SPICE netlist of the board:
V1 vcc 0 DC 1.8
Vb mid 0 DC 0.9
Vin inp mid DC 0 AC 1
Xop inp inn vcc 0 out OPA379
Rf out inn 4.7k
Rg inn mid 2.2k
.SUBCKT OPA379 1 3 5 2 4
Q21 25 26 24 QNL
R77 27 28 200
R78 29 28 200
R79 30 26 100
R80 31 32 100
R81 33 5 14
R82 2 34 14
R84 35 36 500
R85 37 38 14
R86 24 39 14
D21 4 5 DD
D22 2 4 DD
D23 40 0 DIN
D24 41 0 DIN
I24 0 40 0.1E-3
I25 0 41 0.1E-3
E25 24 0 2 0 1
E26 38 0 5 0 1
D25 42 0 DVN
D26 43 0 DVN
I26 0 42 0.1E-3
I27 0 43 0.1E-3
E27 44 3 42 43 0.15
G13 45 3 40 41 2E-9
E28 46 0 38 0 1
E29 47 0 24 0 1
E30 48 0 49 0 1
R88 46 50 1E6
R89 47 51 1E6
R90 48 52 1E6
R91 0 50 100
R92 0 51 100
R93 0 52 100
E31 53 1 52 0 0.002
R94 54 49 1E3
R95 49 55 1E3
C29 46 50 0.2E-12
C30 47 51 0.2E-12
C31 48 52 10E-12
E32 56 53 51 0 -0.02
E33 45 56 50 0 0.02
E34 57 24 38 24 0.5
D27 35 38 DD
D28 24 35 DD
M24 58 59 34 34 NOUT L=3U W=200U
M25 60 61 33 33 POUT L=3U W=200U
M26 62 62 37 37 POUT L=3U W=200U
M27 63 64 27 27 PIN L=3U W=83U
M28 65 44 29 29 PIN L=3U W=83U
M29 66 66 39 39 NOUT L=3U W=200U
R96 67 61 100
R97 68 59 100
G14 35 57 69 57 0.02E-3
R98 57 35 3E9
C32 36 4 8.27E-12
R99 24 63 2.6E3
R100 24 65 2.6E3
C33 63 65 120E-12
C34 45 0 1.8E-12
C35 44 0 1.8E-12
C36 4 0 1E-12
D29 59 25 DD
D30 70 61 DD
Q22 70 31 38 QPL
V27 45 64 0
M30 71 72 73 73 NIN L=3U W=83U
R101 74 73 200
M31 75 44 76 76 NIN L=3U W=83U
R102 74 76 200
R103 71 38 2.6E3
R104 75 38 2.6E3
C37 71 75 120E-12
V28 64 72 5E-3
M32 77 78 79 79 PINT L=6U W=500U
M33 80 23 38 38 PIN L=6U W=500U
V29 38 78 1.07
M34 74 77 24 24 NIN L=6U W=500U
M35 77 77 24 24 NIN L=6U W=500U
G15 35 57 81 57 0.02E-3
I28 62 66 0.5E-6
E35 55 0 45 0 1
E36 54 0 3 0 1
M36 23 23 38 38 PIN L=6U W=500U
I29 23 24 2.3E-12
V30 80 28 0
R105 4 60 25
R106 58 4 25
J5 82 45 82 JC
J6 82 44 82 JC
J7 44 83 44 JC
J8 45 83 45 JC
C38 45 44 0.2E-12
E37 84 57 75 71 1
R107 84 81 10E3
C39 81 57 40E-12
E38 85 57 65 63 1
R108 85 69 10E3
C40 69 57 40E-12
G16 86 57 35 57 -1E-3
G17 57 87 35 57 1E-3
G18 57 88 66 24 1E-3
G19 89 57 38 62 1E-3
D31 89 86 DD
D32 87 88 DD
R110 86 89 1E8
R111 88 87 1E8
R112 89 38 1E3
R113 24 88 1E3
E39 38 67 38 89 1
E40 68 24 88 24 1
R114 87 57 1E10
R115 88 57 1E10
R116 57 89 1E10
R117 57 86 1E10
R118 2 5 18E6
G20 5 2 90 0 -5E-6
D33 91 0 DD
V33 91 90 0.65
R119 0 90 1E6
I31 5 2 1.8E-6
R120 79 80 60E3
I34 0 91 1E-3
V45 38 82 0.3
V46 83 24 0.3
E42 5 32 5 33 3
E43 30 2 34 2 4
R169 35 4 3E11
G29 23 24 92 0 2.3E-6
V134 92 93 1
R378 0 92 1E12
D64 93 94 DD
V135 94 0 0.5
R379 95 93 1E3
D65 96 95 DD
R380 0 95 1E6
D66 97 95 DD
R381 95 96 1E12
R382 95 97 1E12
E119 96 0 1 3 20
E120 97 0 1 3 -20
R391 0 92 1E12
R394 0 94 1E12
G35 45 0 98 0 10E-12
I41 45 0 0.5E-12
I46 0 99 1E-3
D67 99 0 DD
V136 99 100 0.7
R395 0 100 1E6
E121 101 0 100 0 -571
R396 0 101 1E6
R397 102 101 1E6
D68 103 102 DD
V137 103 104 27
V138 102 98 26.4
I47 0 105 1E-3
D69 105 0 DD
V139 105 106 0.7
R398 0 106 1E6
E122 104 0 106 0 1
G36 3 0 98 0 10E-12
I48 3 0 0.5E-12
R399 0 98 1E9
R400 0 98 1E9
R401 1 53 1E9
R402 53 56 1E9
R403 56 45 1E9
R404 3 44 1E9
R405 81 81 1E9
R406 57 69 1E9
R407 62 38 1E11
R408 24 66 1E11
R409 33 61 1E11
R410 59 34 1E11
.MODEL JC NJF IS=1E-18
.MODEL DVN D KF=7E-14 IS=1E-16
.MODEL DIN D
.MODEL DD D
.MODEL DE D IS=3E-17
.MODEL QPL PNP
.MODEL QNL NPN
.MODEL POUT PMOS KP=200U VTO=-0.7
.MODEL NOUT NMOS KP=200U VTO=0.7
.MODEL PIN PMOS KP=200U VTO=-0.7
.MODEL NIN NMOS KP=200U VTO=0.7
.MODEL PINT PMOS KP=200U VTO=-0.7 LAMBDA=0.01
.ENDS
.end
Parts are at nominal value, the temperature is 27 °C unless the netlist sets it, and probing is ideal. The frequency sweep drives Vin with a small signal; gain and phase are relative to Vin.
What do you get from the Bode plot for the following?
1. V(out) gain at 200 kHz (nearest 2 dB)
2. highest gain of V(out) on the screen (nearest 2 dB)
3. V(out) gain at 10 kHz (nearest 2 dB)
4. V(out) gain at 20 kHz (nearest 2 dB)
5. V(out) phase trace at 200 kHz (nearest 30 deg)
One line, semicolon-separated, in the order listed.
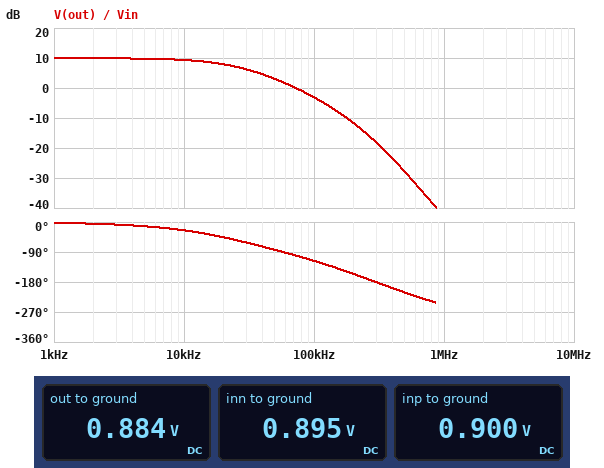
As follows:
-12 dB; 10 dB; 10 dB; 8 dB; -150 deg
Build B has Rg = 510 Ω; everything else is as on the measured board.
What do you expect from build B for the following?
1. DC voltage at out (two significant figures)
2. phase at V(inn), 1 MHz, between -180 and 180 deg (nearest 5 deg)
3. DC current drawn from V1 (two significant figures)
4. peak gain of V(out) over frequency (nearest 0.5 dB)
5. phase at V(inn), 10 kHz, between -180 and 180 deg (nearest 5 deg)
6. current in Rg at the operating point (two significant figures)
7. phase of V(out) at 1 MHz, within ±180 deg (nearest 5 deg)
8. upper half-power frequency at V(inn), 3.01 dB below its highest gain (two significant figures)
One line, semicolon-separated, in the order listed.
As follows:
850 mV; 105 deg; 1.9 µA; 20.0 dB; -55 deg; 9.8 µA; 120 deg; 8.3 kHz
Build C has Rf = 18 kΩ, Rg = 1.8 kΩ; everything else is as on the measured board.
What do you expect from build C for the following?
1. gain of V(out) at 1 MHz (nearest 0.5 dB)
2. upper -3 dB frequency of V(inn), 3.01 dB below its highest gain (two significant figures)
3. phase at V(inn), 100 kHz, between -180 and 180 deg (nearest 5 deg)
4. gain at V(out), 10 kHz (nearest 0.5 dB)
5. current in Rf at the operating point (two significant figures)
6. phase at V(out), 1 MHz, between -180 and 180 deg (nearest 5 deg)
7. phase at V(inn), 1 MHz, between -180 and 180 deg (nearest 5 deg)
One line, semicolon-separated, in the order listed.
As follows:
-41.0 dB; 9.0 kHz; -125 deg; 17.5 dB; 2.8 µA; 115 deg; 95 deg
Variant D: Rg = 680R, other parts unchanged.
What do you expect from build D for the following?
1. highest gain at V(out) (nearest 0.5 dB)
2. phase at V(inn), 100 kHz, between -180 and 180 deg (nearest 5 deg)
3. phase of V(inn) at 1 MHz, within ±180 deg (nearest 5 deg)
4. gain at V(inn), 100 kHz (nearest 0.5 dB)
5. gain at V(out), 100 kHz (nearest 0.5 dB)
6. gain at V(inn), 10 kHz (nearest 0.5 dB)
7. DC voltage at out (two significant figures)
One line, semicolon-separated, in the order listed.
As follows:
18.0 dB; -120 deg; 105 deg; -20.5 dB; -2.5 dB; -3.0 dB; 860 mV
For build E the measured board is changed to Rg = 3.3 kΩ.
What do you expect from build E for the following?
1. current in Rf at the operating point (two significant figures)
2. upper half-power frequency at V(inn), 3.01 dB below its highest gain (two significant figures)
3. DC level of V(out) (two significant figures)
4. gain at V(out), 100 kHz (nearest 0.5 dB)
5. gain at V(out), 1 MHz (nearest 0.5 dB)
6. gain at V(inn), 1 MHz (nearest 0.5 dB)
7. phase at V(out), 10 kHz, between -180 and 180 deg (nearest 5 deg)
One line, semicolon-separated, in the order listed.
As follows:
1.5 µA; 37 kHz; 890 mV; -2.5 dB; -42.0 dB; -45.0 dB; -20 deg
